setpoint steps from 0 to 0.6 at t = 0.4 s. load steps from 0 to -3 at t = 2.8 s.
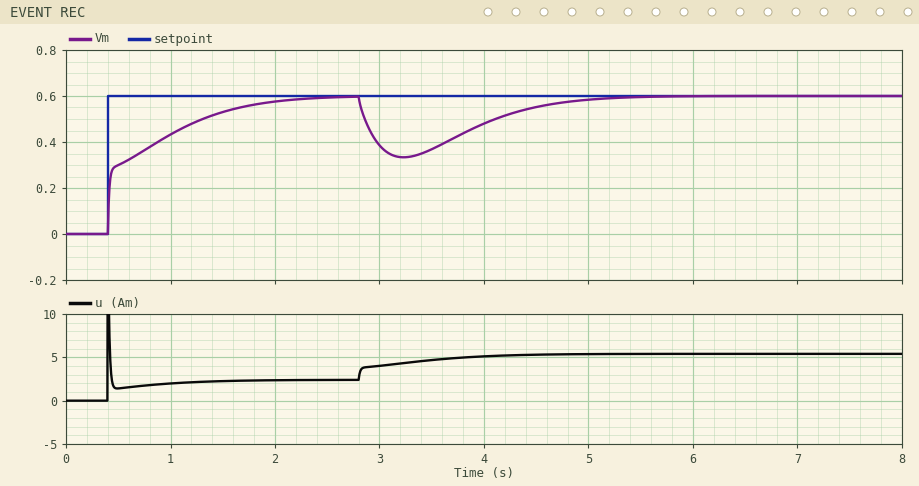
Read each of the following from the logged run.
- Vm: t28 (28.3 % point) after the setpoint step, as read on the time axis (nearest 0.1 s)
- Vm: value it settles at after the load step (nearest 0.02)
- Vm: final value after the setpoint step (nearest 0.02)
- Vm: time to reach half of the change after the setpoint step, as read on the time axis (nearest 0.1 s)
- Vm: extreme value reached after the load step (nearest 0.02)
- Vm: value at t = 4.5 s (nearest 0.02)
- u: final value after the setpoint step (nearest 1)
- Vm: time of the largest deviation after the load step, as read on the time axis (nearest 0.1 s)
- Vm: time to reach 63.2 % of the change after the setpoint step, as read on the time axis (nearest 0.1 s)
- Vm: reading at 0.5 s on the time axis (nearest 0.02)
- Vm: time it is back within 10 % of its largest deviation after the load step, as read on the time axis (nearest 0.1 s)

0.4 s
0.60
0.60
0.5 s
0.34
0.56
2
3.2 s
0.8 s
0.30
4.8 s
